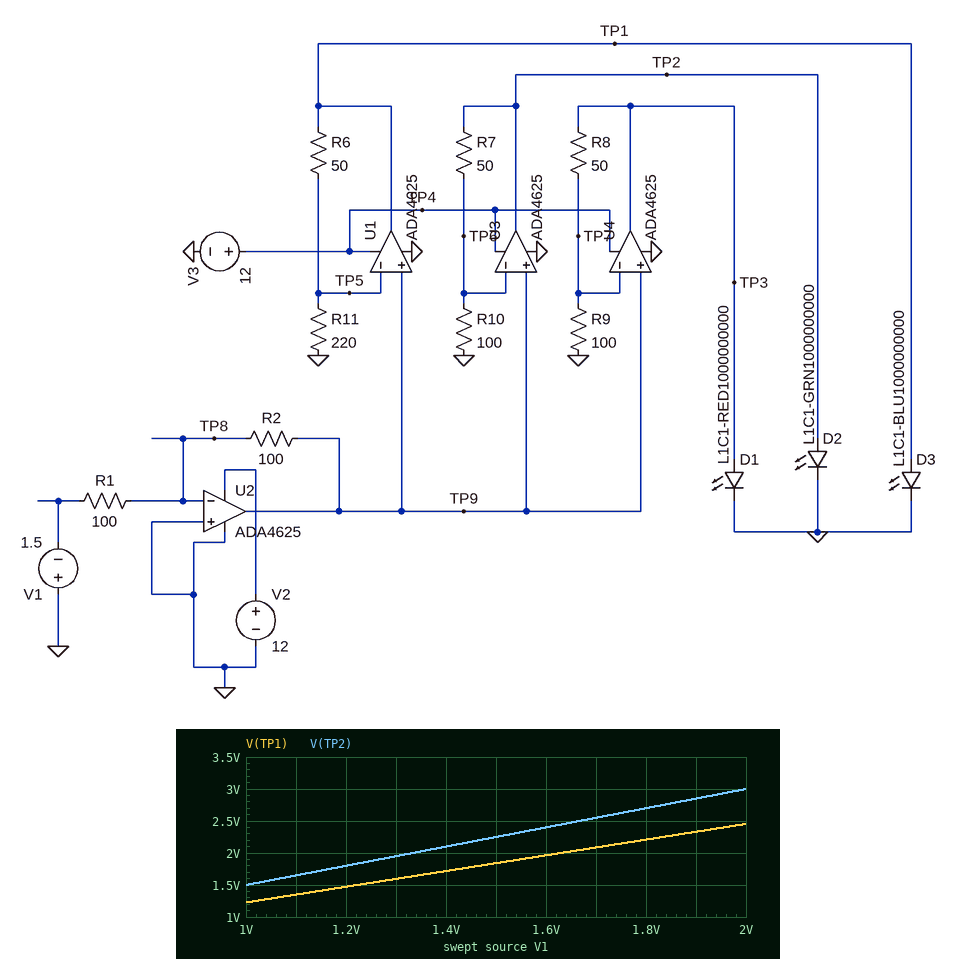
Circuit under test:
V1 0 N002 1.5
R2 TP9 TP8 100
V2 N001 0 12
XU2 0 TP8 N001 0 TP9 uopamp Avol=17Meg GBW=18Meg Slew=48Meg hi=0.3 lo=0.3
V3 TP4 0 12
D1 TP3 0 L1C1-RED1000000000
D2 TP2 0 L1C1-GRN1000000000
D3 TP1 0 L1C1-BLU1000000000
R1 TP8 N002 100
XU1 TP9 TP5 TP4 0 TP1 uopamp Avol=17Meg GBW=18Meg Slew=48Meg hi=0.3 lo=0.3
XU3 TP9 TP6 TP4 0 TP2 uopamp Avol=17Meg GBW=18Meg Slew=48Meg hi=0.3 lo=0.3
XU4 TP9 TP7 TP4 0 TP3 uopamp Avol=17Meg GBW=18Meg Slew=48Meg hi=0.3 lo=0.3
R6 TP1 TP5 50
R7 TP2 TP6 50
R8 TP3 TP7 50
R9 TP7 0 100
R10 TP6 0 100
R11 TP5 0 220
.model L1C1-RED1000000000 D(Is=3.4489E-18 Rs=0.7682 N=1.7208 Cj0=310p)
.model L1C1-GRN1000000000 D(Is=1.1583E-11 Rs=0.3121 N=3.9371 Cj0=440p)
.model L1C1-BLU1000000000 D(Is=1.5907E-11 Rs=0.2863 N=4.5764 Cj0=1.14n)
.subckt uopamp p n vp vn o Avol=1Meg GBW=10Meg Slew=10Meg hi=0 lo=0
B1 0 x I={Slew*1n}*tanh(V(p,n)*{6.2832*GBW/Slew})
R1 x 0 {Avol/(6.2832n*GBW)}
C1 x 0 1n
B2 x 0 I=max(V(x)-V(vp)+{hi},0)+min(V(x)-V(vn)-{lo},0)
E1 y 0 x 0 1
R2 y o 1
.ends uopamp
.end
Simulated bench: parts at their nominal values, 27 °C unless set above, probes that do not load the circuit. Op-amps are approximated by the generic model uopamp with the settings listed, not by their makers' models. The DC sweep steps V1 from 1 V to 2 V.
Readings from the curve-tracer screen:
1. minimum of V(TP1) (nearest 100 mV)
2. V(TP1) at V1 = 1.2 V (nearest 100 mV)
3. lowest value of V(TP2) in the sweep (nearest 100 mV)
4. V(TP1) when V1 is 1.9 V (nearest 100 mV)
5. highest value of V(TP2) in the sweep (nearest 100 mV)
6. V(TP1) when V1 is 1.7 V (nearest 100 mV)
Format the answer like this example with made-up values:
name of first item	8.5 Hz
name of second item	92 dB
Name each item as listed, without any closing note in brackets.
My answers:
minimum of V(TP1)	1.2 V
V(TP1) at V1 = 1.2 V	1.5 V
lowest value of V(TP2) in the sweep	1.5 V
V(TP1) when V1 is 1.9 V	2.3 V
highest value of V(TP2) in the sweep	3.0 V
V(TP1) when V1 is 1.7 V	2.1 V
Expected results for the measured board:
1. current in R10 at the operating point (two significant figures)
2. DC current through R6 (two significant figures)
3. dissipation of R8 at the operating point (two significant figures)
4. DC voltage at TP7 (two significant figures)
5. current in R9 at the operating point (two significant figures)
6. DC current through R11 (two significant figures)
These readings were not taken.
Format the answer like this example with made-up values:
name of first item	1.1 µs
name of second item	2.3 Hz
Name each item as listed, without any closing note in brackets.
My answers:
current in R10 at the operating point	15 mA
DC current through R6	6.8 mA
dissipation of R8 at the operating point	11 mW
DC voltage at TP7	1.5 V
current in R9 at the operating point	15 mA
DC current through R11	6.8 mA
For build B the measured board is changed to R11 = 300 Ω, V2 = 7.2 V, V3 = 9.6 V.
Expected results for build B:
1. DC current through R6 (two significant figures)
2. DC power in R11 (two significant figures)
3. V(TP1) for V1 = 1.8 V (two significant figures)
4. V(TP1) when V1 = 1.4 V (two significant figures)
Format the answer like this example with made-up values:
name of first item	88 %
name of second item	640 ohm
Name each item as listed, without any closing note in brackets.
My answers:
DC current through R6	5.0 mA
DC power in R11	7.5 mW
V(TP1) for V1 = 1.8 V	2.1 V
V(TP1) when V1 = 1.4 V	1.6 V
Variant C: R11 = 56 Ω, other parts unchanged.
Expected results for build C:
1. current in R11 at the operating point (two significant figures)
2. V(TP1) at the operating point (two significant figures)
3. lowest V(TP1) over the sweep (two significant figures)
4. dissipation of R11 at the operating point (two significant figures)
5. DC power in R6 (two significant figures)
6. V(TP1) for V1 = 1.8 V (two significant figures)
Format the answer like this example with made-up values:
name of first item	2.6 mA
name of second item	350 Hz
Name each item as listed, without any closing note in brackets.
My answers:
current in R11 at the operating point	27 mA
V(TP1) at the operating point	2.8 V
lowest V(TP1) over the sweep	1.9 V
dissipation of R11 at the operating point	40 mW
DC power in R6	36 mW
V(TP1) for V1 = 1.8 V	3.4 V
